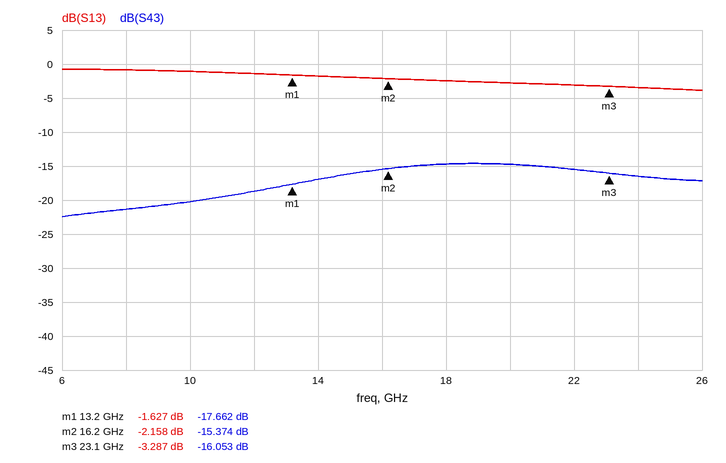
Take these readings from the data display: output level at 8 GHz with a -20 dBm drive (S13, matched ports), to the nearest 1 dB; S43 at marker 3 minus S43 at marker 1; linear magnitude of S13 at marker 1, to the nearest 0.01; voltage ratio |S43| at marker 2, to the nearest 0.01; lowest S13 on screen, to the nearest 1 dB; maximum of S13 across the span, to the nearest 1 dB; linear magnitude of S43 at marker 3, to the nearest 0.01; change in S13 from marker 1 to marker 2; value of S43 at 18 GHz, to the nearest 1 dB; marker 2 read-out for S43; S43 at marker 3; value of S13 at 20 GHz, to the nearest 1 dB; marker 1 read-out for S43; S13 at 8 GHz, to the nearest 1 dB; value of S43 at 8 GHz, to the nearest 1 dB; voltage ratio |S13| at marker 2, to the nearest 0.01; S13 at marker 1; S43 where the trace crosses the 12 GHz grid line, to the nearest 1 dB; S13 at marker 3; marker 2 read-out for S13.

-21 dBm
1.609 dB
0.83
0.17
-4 dB
-1 dB
0.16
-0.531 dB
-15 dB
-15.374 dB
-16.053 dB
-3 dB
-17.662 dB
-1 dB
-21 dB
0.78
-1.627 dB
-19 dB
-3.287 dB
-2.158 dB
